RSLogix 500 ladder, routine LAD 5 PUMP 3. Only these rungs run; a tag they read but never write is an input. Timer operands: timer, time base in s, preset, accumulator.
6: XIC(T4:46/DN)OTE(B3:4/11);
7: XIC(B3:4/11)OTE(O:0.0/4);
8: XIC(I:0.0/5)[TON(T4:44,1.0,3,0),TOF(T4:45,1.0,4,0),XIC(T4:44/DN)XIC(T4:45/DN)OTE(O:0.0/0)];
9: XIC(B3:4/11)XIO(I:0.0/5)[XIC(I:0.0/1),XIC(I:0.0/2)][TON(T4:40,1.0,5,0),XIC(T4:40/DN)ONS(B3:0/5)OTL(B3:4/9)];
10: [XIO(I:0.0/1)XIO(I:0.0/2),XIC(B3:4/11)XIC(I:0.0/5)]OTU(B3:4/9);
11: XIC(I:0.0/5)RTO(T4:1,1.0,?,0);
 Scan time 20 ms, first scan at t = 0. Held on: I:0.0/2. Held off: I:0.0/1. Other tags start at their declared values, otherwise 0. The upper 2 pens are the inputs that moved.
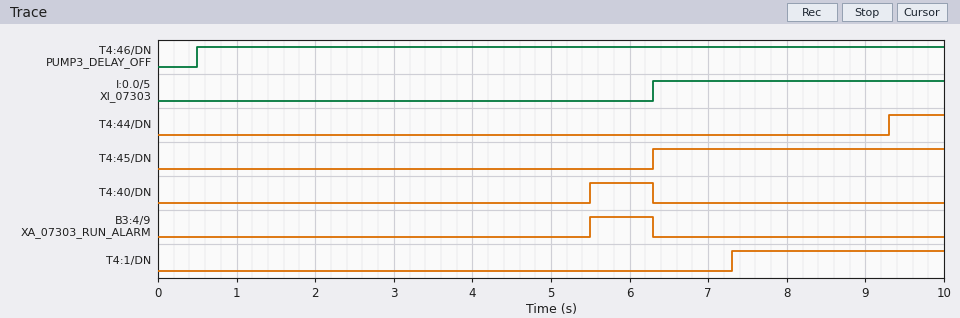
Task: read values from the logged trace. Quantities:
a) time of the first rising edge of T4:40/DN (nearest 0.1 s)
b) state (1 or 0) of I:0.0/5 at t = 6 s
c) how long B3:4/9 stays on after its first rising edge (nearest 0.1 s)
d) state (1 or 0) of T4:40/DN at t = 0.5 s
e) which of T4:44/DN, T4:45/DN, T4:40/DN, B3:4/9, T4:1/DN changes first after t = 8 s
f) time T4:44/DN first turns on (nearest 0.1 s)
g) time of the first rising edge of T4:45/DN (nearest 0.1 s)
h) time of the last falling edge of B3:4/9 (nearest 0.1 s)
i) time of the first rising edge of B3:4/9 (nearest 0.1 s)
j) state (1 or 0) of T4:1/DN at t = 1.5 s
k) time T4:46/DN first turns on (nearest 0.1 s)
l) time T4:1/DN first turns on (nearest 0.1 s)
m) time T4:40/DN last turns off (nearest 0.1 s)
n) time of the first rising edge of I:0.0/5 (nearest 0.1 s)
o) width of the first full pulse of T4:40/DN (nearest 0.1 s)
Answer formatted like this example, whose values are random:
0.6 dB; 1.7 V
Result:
5.5 s; 0; 0.8 s; 0; T4:44/DN; 9.3 s; 6.3 s; 6.3 s; 5.5 s; 0; 0.5 s; 7.3 s; 6.3 s; 6.3 s; 0.8 s
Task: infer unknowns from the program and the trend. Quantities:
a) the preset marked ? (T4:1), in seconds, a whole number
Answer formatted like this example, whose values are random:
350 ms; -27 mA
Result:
1 s
